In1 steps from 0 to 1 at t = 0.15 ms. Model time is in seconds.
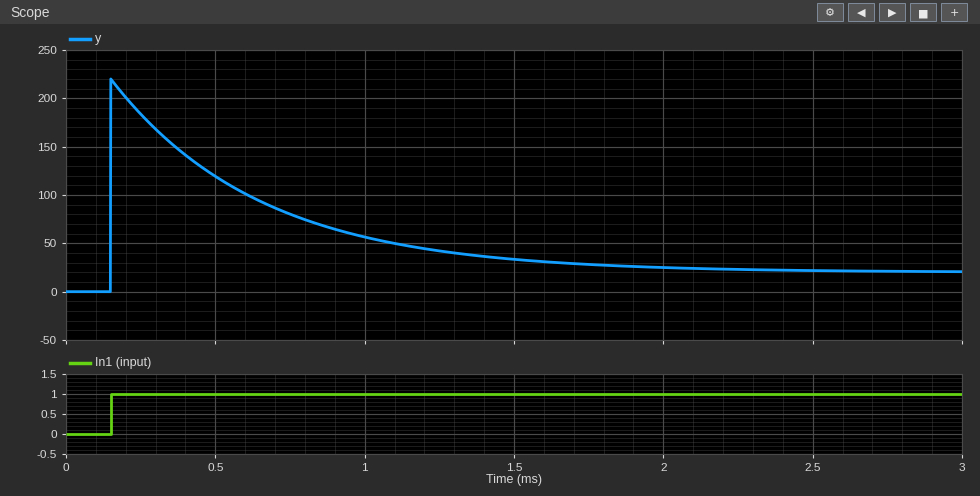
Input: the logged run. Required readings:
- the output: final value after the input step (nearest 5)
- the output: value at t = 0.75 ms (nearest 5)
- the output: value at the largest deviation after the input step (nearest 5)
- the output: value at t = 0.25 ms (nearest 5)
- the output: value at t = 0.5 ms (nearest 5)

20
80
220
185
120
